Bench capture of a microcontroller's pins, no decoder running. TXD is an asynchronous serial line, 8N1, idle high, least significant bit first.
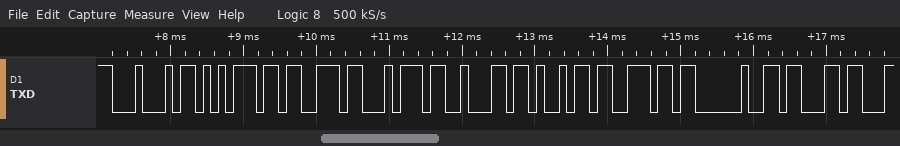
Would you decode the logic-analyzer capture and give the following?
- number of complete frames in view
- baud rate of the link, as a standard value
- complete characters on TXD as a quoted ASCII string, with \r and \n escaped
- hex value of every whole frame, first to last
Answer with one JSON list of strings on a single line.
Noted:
["9", "9600 baud", "\"Dustbin c\"", "0x44 0x75 0x73 0x74 0x62 0x69 0x6E 0x20 0x63"]
